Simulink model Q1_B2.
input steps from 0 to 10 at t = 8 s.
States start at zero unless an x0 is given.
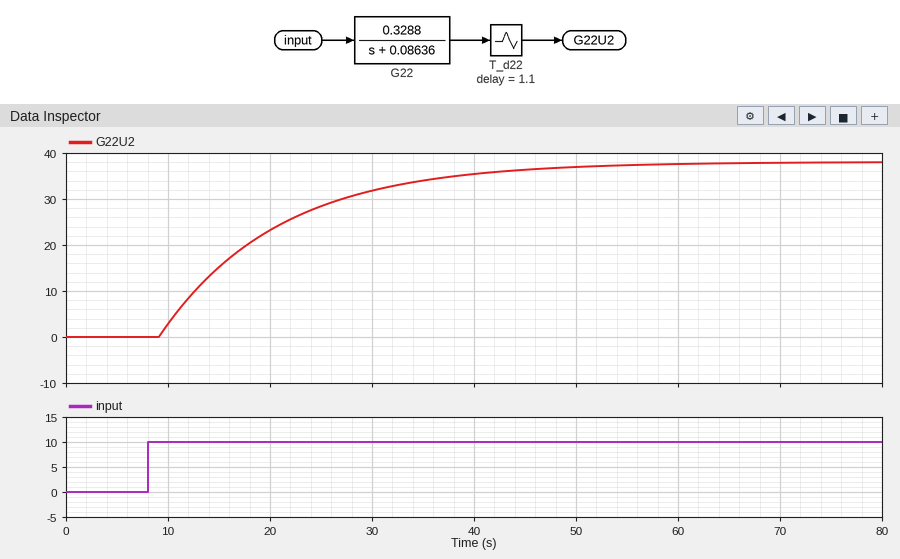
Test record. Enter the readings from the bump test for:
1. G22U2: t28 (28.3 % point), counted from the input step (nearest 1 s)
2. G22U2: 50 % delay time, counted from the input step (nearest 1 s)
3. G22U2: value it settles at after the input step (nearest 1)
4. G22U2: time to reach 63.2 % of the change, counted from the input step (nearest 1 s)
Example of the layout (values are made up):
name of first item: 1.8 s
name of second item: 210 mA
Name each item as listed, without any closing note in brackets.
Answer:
G22U2: t28 (28.3 % point), counted from the input step: 5 s
G22U2: 50 % delay time, counted from the input step: 9 s
G22U2: value it settles at after the input step: 38
G22U2: time to reach 63.2 % of the change, counted from the input step: 13 s
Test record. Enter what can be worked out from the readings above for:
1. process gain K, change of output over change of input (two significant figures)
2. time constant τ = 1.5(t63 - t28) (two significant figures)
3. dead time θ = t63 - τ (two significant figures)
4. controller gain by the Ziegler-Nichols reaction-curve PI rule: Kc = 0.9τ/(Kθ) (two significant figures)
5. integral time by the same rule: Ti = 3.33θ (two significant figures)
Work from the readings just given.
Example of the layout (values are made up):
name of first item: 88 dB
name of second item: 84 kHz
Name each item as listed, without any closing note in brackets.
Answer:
process gain K, change of output over change of input: 3.8
time constant τ = 1.5(t63 - t28): 12 s
dead time θ = t63 - τ: 1.0 s
controller gain by the Ziegler-Nichols reaction-curve PI rule: Kc = 0.9τ/(Kθ): 2.8
integral time by the same rule: Ti = 3.33θ: 3.3 s
